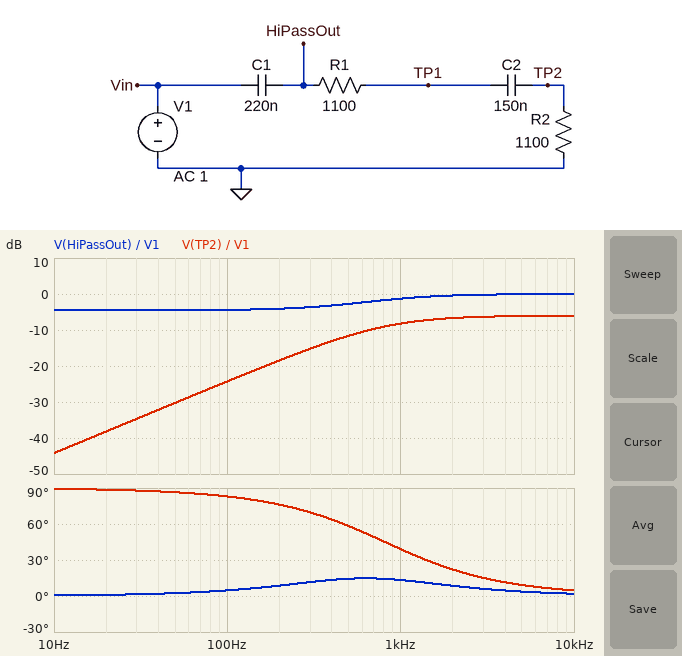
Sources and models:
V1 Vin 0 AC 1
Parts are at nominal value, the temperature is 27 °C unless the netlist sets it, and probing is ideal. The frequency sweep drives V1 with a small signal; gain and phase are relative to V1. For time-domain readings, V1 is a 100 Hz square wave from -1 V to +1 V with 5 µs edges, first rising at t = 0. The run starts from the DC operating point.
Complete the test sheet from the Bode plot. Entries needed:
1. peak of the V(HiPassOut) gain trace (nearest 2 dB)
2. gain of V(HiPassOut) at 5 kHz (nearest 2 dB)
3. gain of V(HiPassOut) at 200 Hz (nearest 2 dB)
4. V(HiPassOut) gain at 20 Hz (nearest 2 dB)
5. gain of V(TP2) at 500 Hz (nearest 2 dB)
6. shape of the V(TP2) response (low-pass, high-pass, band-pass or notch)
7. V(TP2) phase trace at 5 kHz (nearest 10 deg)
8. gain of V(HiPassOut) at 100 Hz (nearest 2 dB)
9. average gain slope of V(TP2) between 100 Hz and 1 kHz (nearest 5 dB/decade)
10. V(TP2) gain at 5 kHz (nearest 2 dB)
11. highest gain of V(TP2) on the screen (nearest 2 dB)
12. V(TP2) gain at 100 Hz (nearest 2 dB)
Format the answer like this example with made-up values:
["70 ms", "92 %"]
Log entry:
["0 dB", "0 dB", "-4 dB", "-4 dB", "-12 dB", "high-pass", "10 deg", "-4 dB", "15 dB/decade", "-6 dB", "-6 dB", "-24 dB"]
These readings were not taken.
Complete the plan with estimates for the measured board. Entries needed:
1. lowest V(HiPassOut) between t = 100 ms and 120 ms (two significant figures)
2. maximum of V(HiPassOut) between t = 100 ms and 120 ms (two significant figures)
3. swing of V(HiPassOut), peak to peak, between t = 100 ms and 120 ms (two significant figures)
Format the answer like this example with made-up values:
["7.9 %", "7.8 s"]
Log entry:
["-800 mV", "2.0 V", "2.8 V"]
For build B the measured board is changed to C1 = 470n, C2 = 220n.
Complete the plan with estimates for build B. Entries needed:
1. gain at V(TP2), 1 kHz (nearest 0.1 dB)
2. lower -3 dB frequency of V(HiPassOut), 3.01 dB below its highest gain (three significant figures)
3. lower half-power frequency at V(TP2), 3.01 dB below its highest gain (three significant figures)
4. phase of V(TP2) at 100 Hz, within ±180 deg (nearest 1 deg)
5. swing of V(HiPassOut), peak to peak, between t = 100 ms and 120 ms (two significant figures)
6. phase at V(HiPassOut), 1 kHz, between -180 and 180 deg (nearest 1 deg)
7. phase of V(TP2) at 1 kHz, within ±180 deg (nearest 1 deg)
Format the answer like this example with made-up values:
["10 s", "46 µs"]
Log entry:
["-6.9 dB", "130 Hz", "483 Hz", "78 deg", "2.6 V", "8 deg", "26 deg"]
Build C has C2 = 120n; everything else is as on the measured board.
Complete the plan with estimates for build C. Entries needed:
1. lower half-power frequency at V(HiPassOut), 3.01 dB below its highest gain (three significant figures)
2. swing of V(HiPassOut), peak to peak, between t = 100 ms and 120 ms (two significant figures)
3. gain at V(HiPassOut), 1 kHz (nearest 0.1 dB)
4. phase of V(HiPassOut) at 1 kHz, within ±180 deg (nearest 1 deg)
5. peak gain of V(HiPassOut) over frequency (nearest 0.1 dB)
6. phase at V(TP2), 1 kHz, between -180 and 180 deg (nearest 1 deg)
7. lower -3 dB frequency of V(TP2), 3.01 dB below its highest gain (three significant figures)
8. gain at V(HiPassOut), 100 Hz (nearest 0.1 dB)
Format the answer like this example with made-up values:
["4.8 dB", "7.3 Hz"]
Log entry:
["376 Hz", "2.7 V", "-1.4 dB", "12 deg", "0 dB", "43 deg", "932 Hz", "-3.7 dB"]
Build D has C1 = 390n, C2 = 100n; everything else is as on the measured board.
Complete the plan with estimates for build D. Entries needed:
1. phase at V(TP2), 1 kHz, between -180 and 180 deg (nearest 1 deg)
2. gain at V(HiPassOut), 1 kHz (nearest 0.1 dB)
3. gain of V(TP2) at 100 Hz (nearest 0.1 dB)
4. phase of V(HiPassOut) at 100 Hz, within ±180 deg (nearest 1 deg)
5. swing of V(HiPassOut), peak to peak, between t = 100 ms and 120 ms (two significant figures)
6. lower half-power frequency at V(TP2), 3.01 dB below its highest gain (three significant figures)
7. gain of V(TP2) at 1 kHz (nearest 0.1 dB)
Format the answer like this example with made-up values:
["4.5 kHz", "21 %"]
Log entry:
["42 deg", "-0.8 dB", "-25.2 dB", "2 deg", "2.4 V", "909 Hz", "-8.6 dB"]
